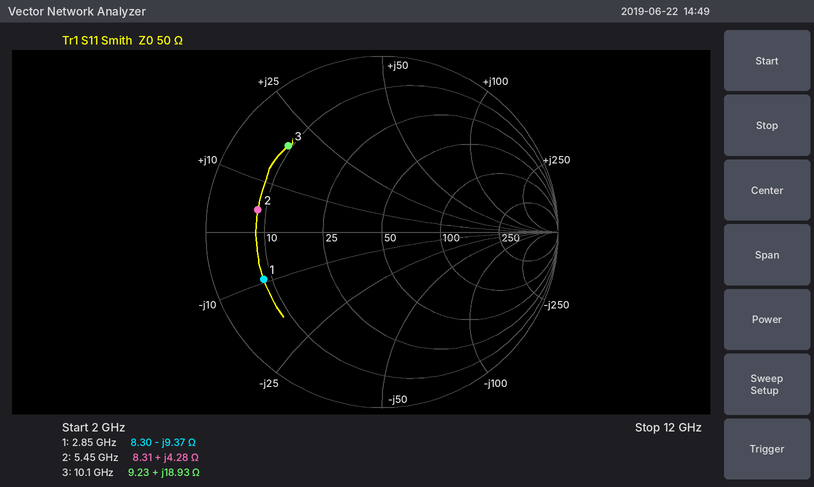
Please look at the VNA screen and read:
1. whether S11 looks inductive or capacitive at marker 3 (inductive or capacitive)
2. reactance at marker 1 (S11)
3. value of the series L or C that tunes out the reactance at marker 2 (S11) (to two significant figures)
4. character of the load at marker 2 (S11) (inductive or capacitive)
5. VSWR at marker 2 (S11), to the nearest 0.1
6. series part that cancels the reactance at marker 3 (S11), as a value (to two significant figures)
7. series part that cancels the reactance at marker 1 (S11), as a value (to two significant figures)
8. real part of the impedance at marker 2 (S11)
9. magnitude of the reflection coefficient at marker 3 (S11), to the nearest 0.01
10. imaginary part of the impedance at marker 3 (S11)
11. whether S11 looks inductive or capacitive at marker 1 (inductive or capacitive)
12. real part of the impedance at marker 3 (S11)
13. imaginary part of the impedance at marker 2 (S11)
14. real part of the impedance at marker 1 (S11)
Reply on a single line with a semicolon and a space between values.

inductive; -9.37 Ω; 6.8 pF; inductive; 6.1; 830 fF; 520 pH; 8.31 Ω; 0.72; +18.93 Ω; capacitive; 9.23 Ω; +4.28 Ω; 8.30 Ω
